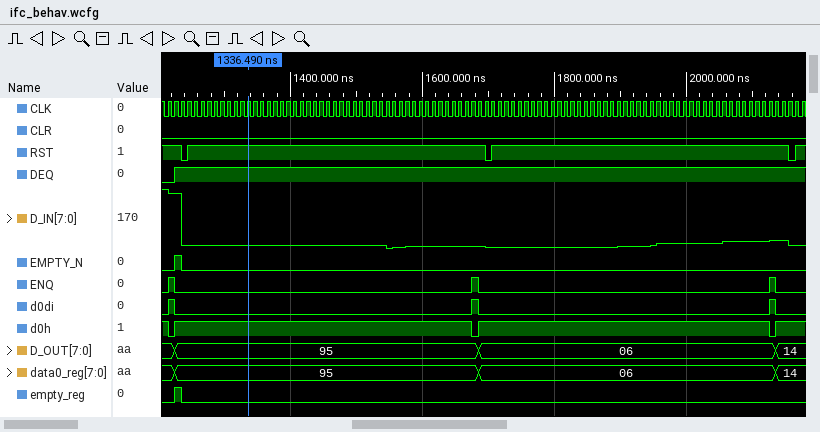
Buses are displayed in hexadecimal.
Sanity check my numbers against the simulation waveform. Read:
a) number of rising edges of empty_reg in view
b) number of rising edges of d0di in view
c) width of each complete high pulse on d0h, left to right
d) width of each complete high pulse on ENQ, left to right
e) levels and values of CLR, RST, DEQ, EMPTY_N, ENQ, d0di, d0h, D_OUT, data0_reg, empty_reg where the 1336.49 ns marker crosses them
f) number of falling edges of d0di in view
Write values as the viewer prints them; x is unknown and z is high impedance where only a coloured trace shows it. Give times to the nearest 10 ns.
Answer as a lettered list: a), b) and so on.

a) 1
b) 3
c) 450 ns, 440 ns
d) 10 ns, 10 ns, 10 ns
e) CLR=0, RST=1, DEQ=1, EMPTY_N=0, ENQ=0, d0di=0, d0h=1, D_OUT=95, data0_reg=95, empty_reg=0
f) 3
